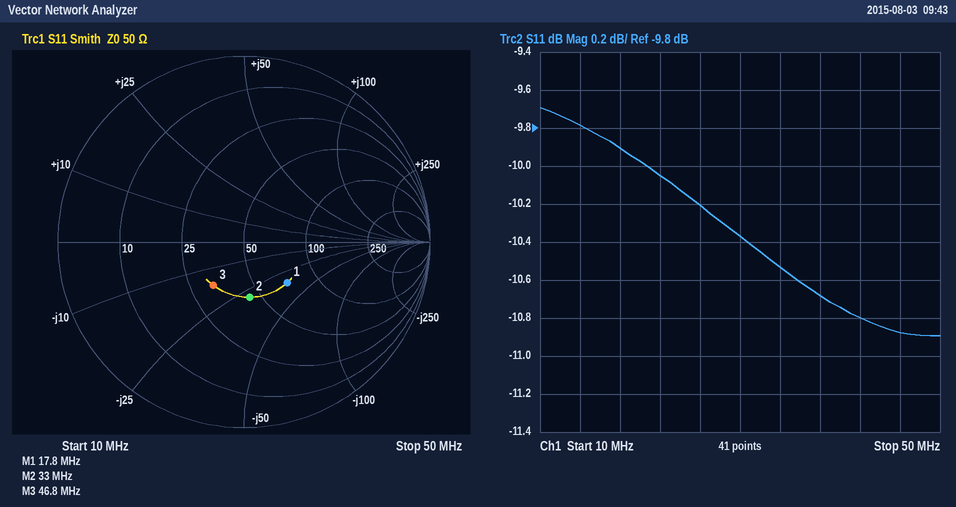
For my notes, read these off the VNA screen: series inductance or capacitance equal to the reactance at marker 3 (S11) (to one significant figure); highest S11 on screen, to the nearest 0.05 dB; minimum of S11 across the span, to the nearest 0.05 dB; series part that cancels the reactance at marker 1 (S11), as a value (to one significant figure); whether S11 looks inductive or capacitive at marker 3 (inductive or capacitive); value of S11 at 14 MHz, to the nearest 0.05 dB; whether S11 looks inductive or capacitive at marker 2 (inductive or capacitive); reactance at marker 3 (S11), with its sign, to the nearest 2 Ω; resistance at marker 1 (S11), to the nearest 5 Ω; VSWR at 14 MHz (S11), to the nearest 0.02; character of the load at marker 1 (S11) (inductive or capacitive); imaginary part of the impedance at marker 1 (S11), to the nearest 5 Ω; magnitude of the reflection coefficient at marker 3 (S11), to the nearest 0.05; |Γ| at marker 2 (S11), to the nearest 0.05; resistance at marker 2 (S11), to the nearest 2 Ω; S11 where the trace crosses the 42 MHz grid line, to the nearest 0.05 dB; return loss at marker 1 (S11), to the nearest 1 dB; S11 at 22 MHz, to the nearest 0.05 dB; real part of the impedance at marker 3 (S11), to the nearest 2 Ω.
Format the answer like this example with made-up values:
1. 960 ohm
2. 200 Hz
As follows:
1. 200 pF
2. -9.70 dB
3. -10.90 dB
4. 300 nH
5. capacitive
6. -9.80 dB
7. capacitive
8. -16 Ω
9. 70 Ω
10. 1.96
11. capacitive
12. -35 Ω
13. 0.30
14. 0.30
15. 44 Ω
16. -10.80 dB
17. 10 dB
18. -10.05 dB
19. 32 Ω
